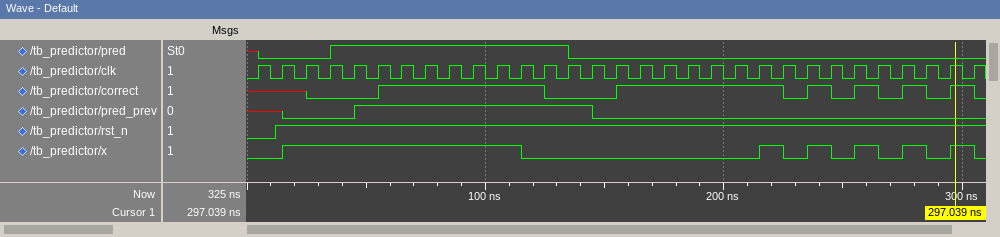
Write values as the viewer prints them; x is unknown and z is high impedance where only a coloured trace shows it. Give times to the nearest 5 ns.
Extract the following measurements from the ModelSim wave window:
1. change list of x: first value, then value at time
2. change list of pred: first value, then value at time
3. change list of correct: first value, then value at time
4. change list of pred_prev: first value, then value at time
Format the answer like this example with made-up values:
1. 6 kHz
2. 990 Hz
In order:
1. 0, 1 at 15 ns, 0 at 115 ns, 1 at 215 ns, 0 at 225 ns, 1 at 235 ns, 0 at 245 ns, 1 at 255 ns, 0 at 265 ns, 1 at 275 ns, 0 at 285 ns, 1 at 295 ns, 0 at 305 ns
2. x, 0 at 5 ns, 1 at 35 ns, 0 at 135 ns
3. x, 0 at 25 ns, 1 at 55 ns, 0 at 125 ns, 1 at 155 ns, 0 at 225 ns, 1 at 235 ns, 0 at 245 ns, 1 at 255 ns, 0 at 265 ns, 1 at 275 ns, 0 at 285 ns, 1 at 295 ns, 0 at 305 ns
4. x, 0 at 15 ns, 1 at 45 ns, 0 at 145 ns
